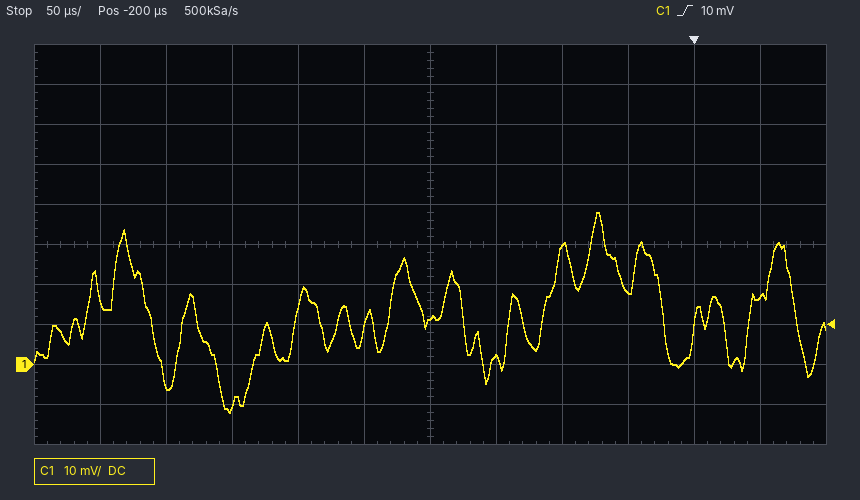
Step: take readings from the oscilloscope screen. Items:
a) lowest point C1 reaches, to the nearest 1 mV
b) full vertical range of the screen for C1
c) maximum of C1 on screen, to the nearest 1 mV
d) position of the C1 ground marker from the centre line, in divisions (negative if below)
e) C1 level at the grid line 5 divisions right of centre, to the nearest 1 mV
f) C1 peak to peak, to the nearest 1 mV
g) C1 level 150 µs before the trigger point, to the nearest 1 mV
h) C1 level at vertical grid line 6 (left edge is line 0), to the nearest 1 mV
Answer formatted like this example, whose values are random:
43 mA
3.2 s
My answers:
-12 mV
100 mV
38 mV
-3.0 div
17 mV
50 mV
2 mV
11 mV
